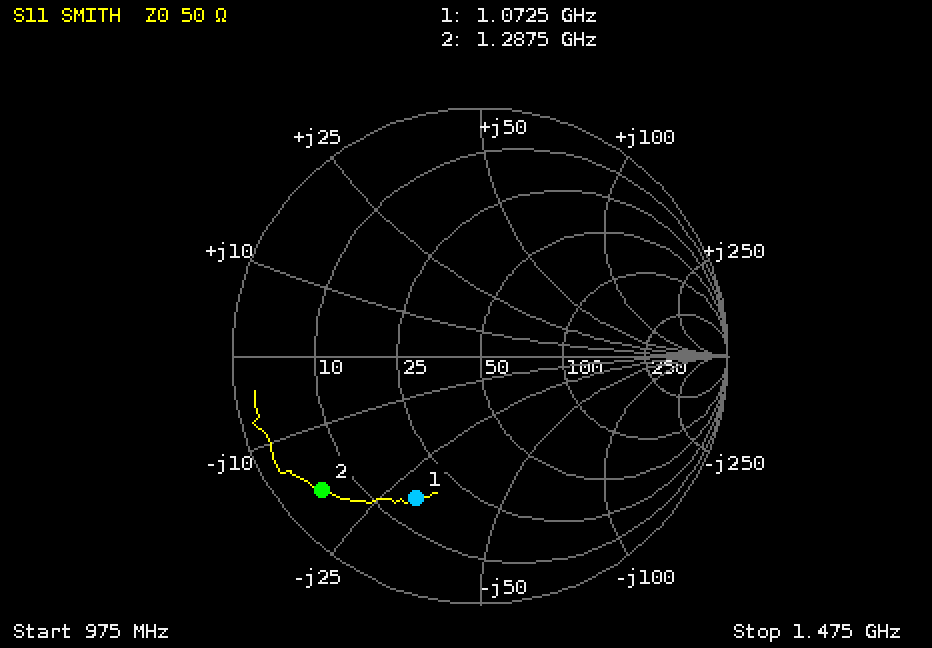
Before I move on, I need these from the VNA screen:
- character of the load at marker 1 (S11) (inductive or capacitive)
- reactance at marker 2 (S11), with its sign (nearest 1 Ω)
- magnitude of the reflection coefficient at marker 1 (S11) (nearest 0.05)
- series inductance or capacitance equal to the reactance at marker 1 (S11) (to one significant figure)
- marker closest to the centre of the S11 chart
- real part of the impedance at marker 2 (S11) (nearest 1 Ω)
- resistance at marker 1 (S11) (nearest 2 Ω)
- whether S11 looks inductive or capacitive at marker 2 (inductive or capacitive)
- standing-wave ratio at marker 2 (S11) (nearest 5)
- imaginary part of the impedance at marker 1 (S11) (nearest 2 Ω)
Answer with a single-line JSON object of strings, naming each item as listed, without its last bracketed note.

{"character of the load at marker 1 (S11)": "capacitive", "reactance at marker 2 (S11), with its sign": "-18 Ω", "magnitude of the reflection coefficient at marker 1 (S11)": "0.65", "series inductance or capacitance equal to the reactance at marker 1 (S11)": "5 pF", "marker closest to the centre of the S11 chart": "marker 1", "real part of the impedance at marker 2 (S11)": "5 Ω", "resistance at marker 1 (S11)": "16 Ω", "whether S11 looks inductive or capacitive at marker 2": "capacitive", "standing-wave ratio at marker 2 (S11)": "10", "imaginary part of the impedance at marker 1 (S11)": "-30 Ω"}
